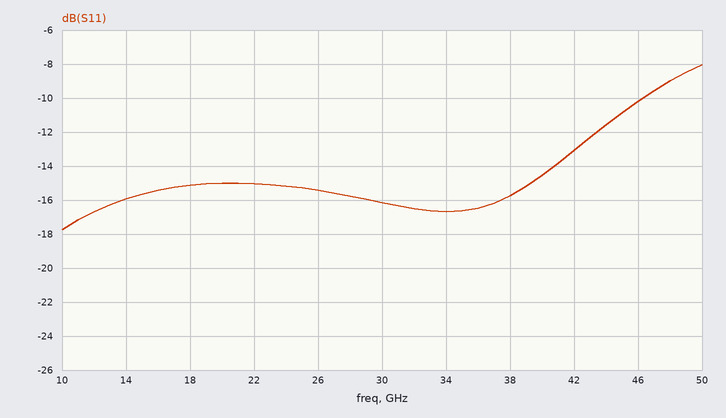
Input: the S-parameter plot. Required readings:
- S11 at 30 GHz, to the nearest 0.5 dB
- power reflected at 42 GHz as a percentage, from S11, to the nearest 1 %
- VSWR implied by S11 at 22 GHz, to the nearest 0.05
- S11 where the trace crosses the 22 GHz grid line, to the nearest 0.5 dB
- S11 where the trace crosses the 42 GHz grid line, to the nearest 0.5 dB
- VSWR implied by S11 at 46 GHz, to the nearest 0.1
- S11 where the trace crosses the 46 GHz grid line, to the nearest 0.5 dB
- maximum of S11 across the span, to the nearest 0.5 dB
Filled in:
-16.0 dB
5 %
1.45
-15.0 dB
-13.0 dB
1.9
-10.0 dB
-8.0 dB
